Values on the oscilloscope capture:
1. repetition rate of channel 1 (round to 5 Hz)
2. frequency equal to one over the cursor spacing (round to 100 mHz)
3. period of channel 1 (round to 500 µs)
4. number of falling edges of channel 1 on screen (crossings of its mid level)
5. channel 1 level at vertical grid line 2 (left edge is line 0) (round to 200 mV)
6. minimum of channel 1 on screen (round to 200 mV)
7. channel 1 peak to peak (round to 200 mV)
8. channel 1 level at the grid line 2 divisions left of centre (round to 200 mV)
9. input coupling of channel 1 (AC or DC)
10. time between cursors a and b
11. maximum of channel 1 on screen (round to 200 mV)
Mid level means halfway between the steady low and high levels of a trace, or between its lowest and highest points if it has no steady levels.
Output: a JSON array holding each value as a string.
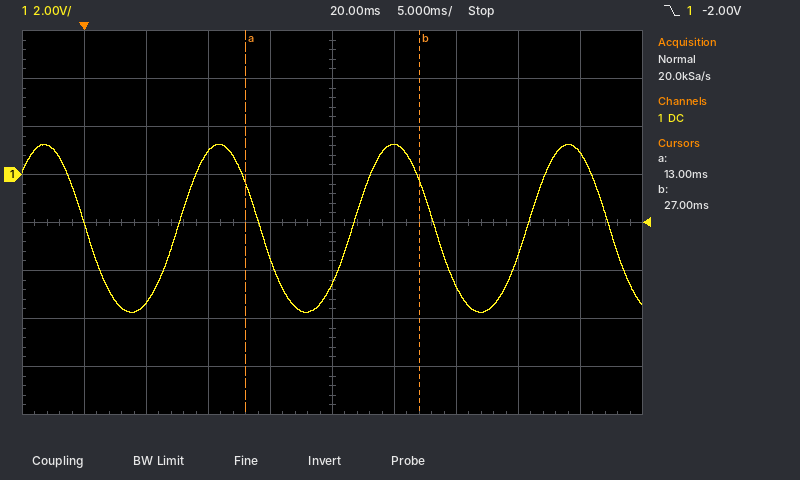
["70 Hz", "71.4 Hz", "14.0 ms", "4", "-5.4 V", "-5.8 V", "7.0 V", "1.0 V", "DC", "14.0 ms", "1.2 V"]
